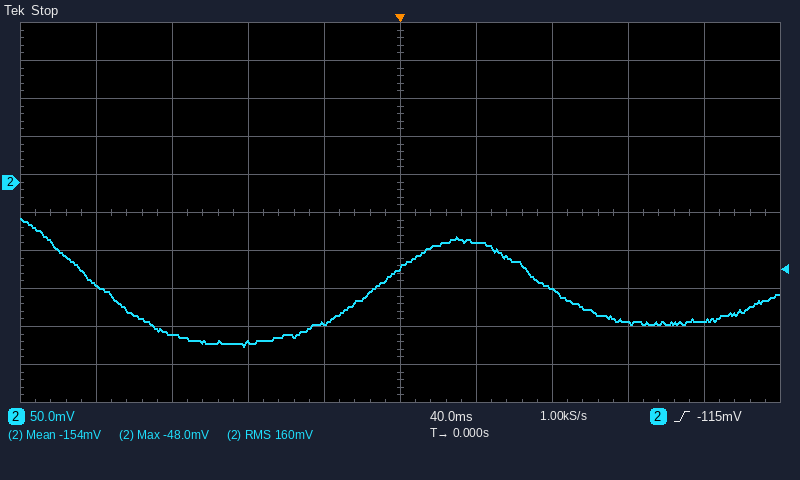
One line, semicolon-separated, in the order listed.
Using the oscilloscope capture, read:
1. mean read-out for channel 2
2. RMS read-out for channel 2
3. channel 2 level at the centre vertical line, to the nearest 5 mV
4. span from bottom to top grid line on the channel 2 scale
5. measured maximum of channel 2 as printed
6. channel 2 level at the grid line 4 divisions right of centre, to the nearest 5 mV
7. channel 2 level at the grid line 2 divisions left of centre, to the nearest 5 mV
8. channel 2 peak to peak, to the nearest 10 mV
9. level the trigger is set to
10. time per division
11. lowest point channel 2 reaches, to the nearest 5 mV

-154 mV; 160 mV; -110 mV; 500 mV; -48.0 mV; -180 mV; -210 mV; 170 mV; -115 mV; 40 ms; -215 mV
